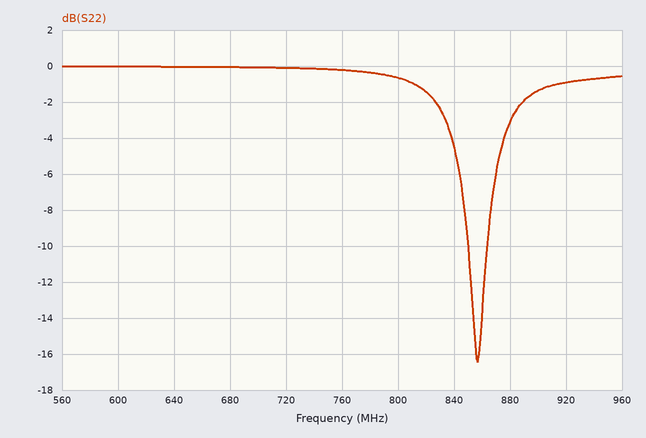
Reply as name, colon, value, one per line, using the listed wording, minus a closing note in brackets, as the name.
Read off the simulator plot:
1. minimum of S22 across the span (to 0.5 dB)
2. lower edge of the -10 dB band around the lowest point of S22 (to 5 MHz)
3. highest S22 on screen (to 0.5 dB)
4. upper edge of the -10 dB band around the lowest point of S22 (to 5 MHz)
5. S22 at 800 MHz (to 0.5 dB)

minimum of S22 across the span: -16.5 dB
lower edge of the -10 dB band around the lowest point of S22: 850 MHz
highest S22 on screen: 0.0 dB
upper edge of the -10 dB band around the lowest point of S22: 865 MHz
S22 at 800 MHz: -0.5 dB
